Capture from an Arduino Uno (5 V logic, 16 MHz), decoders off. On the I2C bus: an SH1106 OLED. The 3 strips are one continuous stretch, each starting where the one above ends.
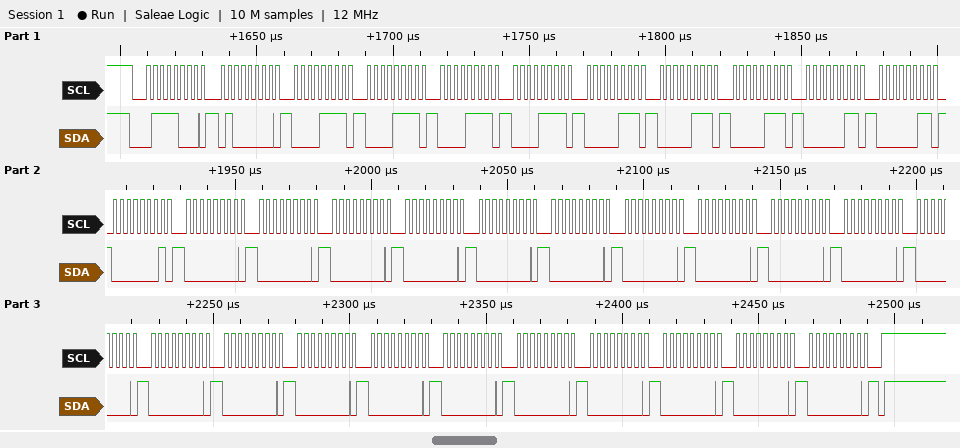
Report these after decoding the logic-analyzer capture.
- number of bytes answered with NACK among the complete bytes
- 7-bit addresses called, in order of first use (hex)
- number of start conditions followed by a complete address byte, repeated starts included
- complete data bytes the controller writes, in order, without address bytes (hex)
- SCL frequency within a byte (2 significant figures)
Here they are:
0
0x3C
1
40 0F 0F 0F 0F 07 07 07 03 03 01 00 00 00 00 00 00 00 00 00 00 00 00 00 00 00 00 00 00 00 00 00
400 kHz
